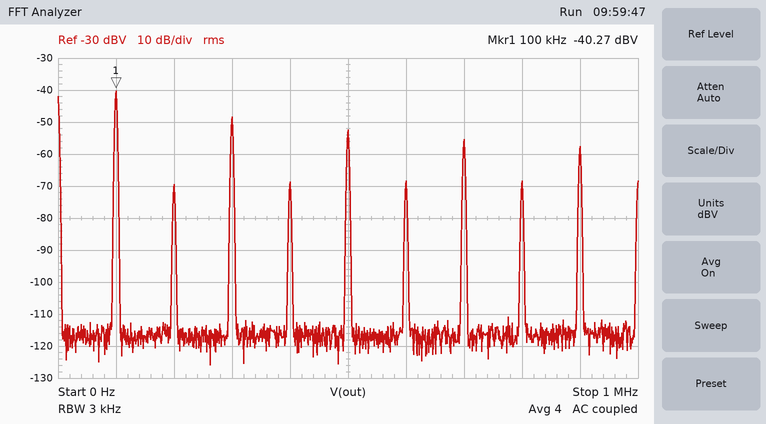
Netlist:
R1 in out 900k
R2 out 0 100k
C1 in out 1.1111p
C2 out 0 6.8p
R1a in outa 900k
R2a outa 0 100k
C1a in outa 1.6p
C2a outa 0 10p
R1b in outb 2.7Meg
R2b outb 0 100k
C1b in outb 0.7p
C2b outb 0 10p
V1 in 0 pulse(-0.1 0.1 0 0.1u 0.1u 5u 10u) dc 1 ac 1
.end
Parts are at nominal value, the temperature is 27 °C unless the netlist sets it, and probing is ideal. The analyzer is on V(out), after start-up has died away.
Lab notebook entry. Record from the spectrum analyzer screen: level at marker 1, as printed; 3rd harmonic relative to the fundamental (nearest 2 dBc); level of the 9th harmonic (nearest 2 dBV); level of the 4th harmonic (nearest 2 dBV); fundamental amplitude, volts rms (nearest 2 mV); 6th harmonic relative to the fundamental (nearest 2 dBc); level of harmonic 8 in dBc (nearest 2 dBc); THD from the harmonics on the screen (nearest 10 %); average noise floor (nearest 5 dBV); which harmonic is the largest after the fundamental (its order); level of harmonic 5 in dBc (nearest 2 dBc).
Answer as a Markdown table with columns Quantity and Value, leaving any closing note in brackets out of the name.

| Quantity | Value |
|---|---|
| level at marker 1, as printed | -40.27 dBV |
| 3rd harmonic relative to the fundamental | -8 dBc |
| level of the 9th harmonic | -58 dBV |
| level of the 4th harmonic | -68 dBV |
| fundamental amplitude, volts rms | 10 mV |
| 6th harmonic relative to the fundamental | -28 dBc |
| level of harmonic 8 in dBc | -28 dBc |
| THD from the harmonics on the screen | 50 % |
| average noise floor | -115 dBV |
| which harmonic is the largest after the fundamental | 3 |
| level of harmonic 5 in dBc | -12 dBc |
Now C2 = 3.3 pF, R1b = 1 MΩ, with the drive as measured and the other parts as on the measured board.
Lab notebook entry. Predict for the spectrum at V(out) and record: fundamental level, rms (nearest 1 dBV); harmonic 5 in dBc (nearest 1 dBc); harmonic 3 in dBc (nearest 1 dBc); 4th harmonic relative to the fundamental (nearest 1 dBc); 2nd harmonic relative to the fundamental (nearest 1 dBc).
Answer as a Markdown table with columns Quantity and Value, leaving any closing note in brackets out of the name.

| Quantity | Value |
|---|---|
| fundamental level, rms | -40 dBV |
| harmonic 5 in dBc | -9 dBc |
| harmonic 3 in dBc | -6 dBc |
| 4th harmonic relative to the fundamental | -26 dBc |
| 2nd harmonic relative to the fundamental | -28 dBc |
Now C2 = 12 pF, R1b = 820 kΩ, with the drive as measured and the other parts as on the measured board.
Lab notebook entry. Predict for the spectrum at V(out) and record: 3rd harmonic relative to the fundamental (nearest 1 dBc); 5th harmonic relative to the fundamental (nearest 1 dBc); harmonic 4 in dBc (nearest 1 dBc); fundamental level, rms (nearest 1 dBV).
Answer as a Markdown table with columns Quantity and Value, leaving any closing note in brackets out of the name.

| Quantity | Value |
|---|---|
| 3rd harmonic relative to the fundamental | -10 dBc |
| 5th harmonic relative to the fundamental | -15 dBc |
| harmonic 4 in dBc | -31 dBc |
| fundamental level, rms | -41 dBV |
